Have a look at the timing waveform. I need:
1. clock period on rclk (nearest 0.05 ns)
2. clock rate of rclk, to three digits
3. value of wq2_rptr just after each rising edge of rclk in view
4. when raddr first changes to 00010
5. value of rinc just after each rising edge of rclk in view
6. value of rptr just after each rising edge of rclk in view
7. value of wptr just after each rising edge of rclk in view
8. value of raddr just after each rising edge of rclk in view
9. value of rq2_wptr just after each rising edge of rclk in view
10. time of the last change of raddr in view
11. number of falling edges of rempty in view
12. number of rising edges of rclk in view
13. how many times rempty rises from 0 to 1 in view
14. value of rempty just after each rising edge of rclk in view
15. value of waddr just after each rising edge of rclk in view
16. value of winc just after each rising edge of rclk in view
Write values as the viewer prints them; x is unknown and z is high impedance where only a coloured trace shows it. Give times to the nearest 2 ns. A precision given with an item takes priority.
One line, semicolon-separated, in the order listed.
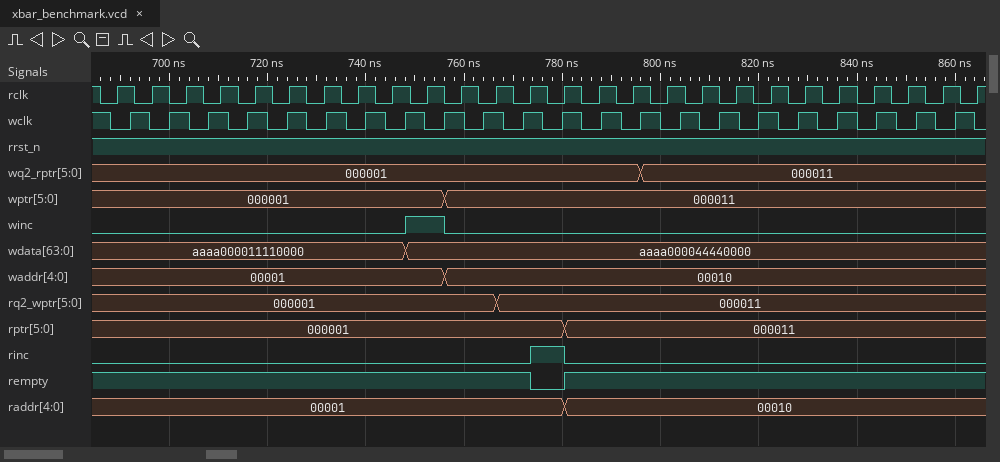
7 ns; 143 MHz; 000001, 000001, 000001, 000001, 000001, 000001, 000001, 000001, 000001, 000001, 000001, 000001, 000001, 000001, 000001, 000001, 000011, 000011, 000011, 000011, 000011, 000011, 000011, 000011, 000011, 000011; 780 ns; 0 0 0 0 0 0 0 0 0 0 0 0 1 0 0 0 0 0 0 0 0 0 0 0 0 0; 000001, 000001, 000001, 000001, 000001, 000001, 000001, 000001, 000001, 000001, 000001, 000001, 000001, 000011, 000011, 000011, 000011, 000011, 000011, 000011, 000011, 000011, 000011, 000011, 000011, 000011; 000001, 000001, 000001, 000001, 000001, 000001, 000001, 000001, 000001, 000001, 000011, 000011, 000011, 000011, 000011, 000011, 000011, 000011, 000011, 000011, 000011, 000011, 000011, 000011, 000011, 000011; 00001, 00001, 00001, 00001, 00001, 00001, 00001, 00001, 00001, 00001, 00001, 00001, 00001, 00010, 00010, 00010, 00010, 00010, 00010, 00010, 00010, 00010, 00010, 00010, 00010, 00010; 000001, 000001, 000001, 000001, 000001, 000001, 000001, 000001, 000001, 000001, 000001, 000011, 000011, 000011, 000011, 000011, 000011, 000011, 000011, 000011, 000011, 000011, 000011, 000011, 000011, 000011; 780 ns; 1; 26; 1; 1 1 1 1 1 1 1 1 1 1 1 1 0 1 1 1 1 1 1 1 1 1 1 1 1 1; 00001, 00001, 00001, 00001, 00001, 00001, 00001, 00001, 00001, 00001, 00010, 00010, 00010, 00010, 00010, 00010, 00010, 00010, 00010, 00010, 00010, 00010, 00010, 00010, 00010, 00010; 0 0 0 0 0 0 0 0 0 1 0 0 0 0 0 0 0 0 0 0 0 0 0 0 0 0
